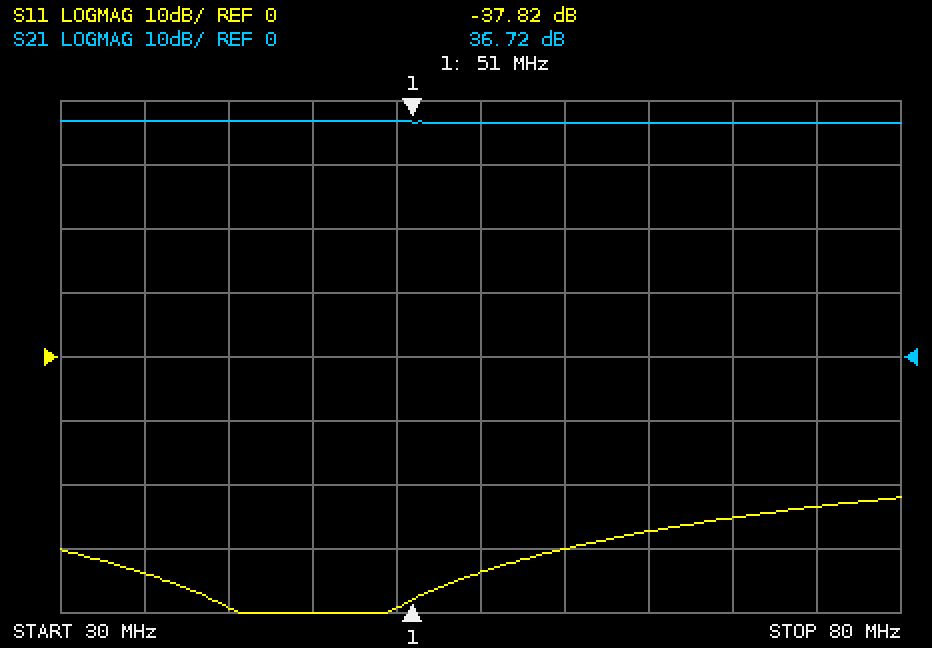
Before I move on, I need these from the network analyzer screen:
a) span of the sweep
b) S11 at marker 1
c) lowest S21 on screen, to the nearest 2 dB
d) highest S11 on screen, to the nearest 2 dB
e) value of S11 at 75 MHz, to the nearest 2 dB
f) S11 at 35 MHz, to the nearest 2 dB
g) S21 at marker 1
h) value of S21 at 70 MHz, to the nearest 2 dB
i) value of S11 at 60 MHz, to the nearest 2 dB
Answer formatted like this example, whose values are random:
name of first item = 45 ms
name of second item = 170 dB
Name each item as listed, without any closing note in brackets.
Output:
span of the sweep = 50 MHz
S11 at marker 1 = -37.82 dB
lowest S21 on screen, to the nearest 2 dB = 36 dB
highest S11 on screen, to the nearest 2 dB = -22 dB
value of S11 at 75 MHz, to the nearest 2 dB = -24 dB
S11 at 35 MHz, to the nearest 2 dB = -34 dB
S21 at marker 1 = 36.72 dB
value of S21 at 70 MHz, to the nearest 2 dB = 36 dB
value of S11 at 60 MHz, to the nearest 2 dB = -30 dB
